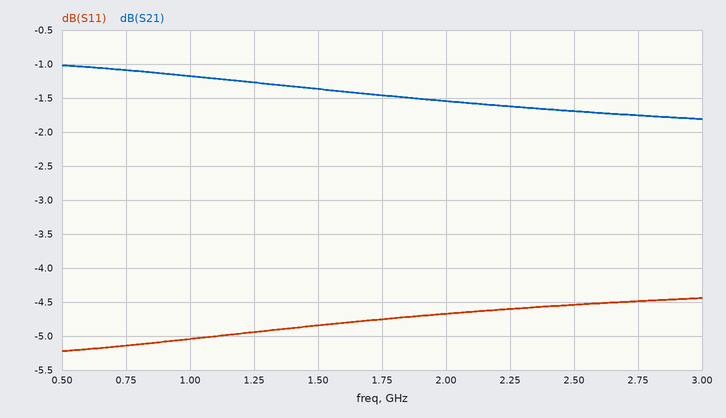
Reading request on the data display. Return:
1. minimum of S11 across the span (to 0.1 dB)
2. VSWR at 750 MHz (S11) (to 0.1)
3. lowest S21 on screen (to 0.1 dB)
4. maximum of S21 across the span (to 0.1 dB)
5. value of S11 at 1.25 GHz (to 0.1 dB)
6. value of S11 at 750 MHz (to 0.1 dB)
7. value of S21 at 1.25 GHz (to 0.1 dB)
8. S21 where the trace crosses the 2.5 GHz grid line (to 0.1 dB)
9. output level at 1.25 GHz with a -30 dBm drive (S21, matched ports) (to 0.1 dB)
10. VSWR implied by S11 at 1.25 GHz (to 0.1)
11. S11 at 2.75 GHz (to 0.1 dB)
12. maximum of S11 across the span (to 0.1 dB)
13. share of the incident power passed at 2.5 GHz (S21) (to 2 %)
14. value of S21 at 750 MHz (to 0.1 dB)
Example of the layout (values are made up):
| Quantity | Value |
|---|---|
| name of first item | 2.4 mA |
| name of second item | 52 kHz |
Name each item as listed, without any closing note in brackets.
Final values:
| Quantity | Value |
|---|---|
| minimum of S11 across the span | -5.2 dB |
| VSWR at 750 MHz (S11) | 3.5 |
| lowest S21 on screen | -1.8 dB |
| maximum of S21 across the span | -1.0 dB |
| value of S11 at 1.25 GHz | -4.9 dB |
| value of S11 at 750 MHz | -5.1 dB |
| value of S21 at 1.25 GHz | -1.3 dB |
| S21 where the trace crosses the 2.5 GHz grid line | -1.7 dB |
| output level at 1.25 GHz with a -30 dBm drive (S21, matched ports) | -31.3 dBm |
| VSWR implied by S11 at 1.25 GHz | 3.6 |
| S11 at 2.75 GHz | -4.5 dB |
| maximum of S11 across the span | -4.4 dB |
| share of the incident power passed at 2.5 GHz (S21) | 68 % |
| value of S21 at 750 MHz | -1.1 dB |
